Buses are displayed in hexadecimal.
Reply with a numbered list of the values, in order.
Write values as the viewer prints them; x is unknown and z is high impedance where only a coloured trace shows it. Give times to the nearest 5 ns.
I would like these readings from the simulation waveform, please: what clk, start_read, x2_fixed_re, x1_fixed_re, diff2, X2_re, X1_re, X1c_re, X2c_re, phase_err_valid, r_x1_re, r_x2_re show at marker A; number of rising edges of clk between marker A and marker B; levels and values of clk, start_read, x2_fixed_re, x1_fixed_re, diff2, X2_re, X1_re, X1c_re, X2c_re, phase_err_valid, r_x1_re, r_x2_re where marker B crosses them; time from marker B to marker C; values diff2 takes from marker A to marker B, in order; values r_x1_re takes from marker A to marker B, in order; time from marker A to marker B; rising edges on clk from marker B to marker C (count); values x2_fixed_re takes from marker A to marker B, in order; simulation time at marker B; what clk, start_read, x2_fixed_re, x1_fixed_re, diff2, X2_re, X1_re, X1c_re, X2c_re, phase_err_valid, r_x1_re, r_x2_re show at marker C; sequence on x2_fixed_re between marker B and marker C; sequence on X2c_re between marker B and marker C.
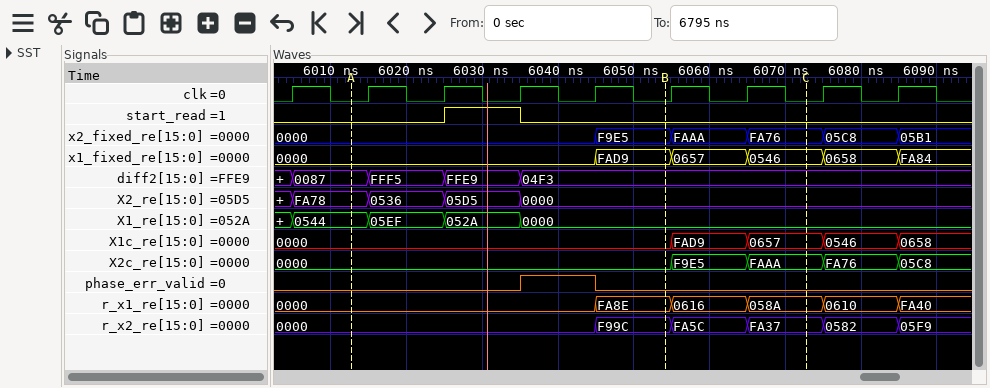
1. clk=0, start_read=0, x2_fixed_re=0000, x1_fixed_re=0000, diff2=0087, X2_re=FA78, X1_re=0544, X1c_re=0000, X2c_re=0000, phase_err_valid=0, r_x1_re=0000, r_x2_re=0000
2. 4
3. clk=0, start_read=0, x2_fixed_re=F9E5, x1_fixed_re=FAD9, diff2=04F3, X2_re=0000, X1_re=0000, X1c_re=0000, X2c_re=0000, phase_err_valid=0, r_x1_re=FA8E, r_x2_re=F99C
4. 20 ns
5. 0087, FFF5, FFE9, 04F3
6. 0000, FA8E
7. 40 ns
8. 2
9. 0000, F9E5
10. 6055 ns
11. clk=0, start_read=0, x2_fixed_re=FA76, x1_fixed_re=0546, diff2=04F3, X2_re=0000, X1_re=0000, X1c_re=0657, X2c_re=FAAA, phase_err_valid=0, r_x1_re=058A, r_x2_re=FA37
12. F9E5, FAAA, FA76
13. 0000, F9E5, FAAA
